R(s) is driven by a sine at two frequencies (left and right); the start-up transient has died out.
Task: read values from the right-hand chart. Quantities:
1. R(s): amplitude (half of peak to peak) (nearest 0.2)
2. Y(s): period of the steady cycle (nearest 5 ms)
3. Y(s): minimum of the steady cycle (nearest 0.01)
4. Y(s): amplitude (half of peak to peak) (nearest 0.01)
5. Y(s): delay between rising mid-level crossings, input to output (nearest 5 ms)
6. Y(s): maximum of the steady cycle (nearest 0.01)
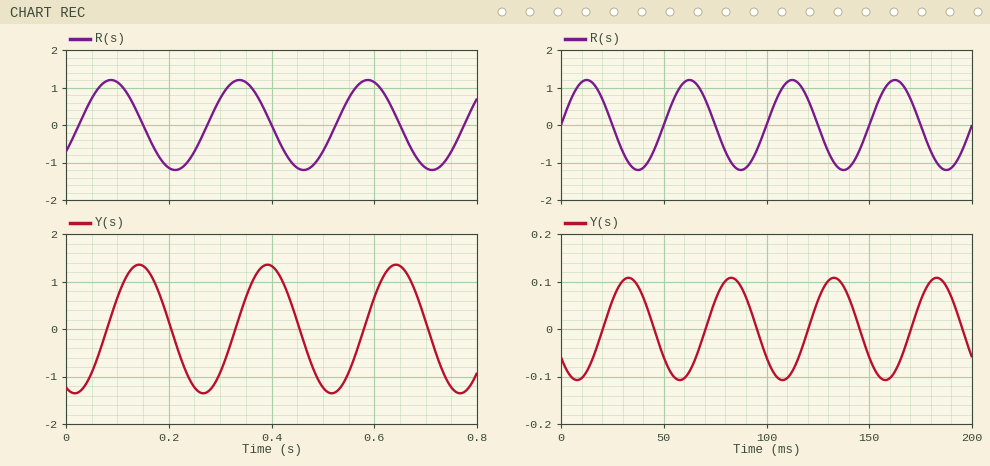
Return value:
1.2
50 ms
-0.11
0.11
20 ms
0.11
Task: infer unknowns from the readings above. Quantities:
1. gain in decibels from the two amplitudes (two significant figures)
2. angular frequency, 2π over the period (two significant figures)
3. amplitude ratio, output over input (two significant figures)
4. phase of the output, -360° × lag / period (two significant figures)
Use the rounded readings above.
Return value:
-21 dB
0.13 rad/ms
0.092
-140°
